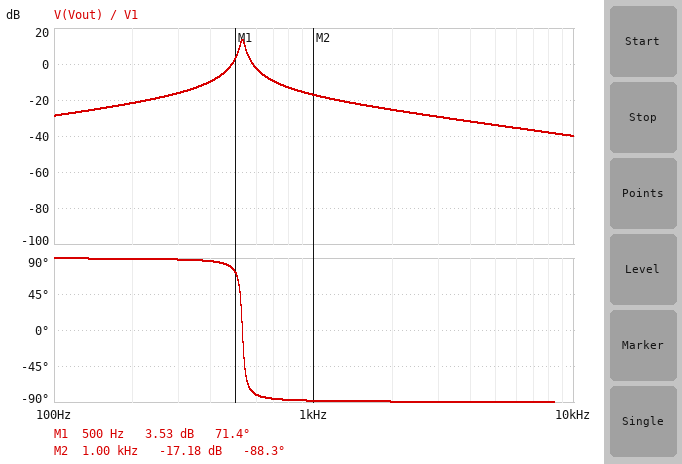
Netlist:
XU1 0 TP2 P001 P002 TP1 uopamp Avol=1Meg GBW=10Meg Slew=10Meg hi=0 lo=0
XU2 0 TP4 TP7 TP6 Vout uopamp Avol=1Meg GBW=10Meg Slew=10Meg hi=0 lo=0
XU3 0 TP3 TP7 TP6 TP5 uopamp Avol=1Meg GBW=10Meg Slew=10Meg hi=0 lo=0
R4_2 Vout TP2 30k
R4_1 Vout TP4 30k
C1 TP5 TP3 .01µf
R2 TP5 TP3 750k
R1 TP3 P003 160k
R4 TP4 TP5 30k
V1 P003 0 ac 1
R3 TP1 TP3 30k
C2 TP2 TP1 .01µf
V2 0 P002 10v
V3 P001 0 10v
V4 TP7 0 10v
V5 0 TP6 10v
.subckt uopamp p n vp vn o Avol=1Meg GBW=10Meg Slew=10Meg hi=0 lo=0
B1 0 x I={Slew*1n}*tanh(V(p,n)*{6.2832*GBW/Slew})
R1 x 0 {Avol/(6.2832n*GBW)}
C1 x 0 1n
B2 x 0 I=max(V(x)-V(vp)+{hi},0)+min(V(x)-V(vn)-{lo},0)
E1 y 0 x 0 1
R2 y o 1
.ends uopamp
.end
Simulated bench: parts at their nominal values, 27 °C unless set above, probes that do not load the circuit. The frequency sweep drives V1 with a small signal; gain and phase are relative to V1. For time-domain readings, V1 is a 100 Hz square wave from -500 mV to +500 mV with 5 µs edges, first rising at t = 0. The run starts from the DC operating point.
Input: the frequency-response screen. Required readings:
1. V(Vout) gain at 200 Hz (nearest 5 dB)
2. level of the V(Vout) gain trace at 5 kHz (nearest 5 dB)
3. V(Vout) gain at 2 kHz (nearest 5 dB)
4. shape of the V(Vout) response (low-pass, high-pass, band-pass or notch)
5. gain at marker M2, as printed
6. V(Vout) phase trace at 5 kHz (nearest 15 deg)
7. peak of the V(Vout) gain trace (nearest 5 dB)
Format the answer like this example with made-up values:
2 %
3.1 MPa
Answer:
-20 dB
-35 dB
-25 dB
band-pass
-17.18 dB
-90 deg
15 dB
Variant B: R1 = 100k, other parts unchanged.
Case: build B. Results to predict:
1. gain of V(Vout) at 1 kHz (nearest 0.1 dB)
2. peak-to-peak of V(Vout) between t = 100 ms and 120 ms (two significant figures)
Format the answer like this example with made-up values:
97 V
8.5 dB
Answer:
-13.1 dB
720 mV
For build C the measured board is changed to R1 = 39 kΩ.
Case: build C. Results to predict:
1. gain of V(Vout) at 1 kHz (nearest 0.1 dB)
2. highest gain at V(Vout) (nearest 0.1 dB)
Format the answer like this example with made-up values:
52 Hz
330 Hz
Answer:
-4.9 dB
25.7 dB
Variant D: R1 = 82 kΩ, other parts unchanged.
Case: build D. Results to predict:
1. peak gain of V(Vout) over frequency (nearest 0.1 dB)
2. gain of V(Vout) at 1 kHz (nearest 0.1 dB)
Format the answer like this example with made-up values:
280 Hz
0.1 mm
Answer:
19.3 dB
-11.4 dB
